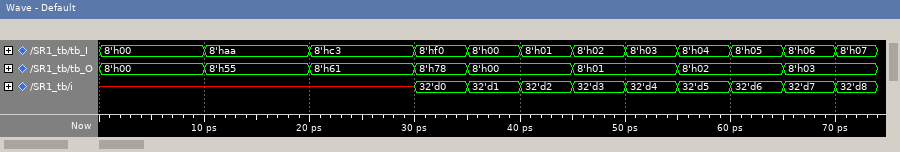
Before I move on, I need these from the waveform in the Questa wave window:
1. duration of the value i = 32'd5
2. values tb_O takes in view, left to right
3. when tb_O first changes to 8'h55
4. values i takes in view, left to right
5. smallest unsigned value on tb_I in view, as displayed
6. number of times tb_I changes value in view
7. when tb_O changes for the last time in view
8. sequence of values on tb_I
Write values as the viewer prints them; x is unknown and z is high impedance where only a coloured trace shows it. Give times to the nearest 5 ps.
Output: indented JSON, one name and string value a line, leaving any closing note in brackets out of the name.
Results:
{
  "duration of the value i = 32'd5": "5 ps",
  "values tb_O takes in view, left to right": "8'h00, 8'h55, 8'h61, 8'h78, 8'h00, 8'h01, 8'h02, 8'h03",
  "when tb_O first changes to 8'h55": "10 ps",
  "values i takes in view, left to right": "x, 32'd0, 32'd1, 32'd2, 32'd3, 32'd4, 32'd5, 32'd6, 32'd7, 32'd8",
  "smallest unsigned value on tb_I in view, as displayed": "8'h00",
  "number of times tb_I changes value in view": "11",
  "when tb_O changes for the last time in view": "65 ps",
  "sequence of values on tb_I": "8'h00, 8'haa, 8'hc3, 8'hf0, 8'h00, 8'h01, 8'h02, 8'h03, 8'h04, 8'h05, 8'h06, 8'h07"
}
